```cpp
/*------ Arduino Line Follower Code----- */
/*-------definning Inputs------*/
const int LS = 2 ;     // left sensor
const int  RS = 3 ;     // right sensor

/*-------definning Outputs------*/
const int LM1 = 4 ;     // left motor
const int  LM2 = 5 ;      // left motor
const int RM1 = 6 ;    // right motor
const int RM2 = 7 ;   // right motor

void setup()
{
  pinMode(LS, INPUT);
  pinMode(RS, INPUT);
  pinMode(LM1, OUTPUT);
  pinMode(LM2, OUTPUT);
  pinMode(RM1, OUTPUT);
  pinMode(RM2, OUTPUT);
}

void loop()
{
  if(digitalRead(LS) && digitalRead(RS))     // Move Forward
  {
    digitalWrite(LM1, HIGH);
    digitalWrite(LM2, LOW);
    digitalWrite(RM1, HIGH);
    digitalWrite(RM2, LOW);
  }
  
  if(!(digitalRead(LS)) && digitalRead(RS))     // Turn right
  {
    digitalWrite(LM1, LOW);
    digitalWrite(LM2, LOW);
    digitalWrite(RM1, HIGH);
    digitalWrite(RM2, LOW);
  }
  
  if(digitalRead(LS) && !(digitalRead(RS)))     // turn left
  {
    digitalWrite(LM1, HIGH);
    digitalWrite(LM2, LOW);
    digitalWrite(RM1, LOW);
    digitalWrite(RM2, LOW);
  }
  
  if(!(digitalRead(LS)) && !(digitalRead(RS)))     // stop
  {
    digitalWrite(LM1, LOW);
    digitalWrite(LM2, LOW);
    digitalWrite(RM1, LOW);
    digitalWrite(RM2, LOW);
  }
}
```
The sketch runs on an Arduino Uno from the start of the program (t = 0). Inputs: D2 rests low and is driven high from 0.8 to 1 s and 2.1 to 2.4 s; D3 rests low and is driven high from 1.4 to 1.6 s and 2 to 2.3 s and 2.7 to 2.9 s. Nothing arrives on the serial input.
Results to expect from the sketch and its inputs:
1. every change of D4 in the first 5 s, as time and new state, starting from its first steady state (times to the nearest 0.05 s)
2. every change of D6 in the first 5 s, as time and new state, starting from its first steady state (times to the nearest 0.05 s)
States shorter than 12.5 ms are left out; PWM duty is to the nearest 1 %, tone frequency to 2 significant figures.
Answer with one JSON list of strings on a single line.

["0 s low; 0.8 s high; 1 s low; 2.1 s high; 2.4 s low", "0 s low; 1.4 s high; 1.6 s low; 2 s high; 2.3 s low; 2.7 s high; 2.9 s low"]
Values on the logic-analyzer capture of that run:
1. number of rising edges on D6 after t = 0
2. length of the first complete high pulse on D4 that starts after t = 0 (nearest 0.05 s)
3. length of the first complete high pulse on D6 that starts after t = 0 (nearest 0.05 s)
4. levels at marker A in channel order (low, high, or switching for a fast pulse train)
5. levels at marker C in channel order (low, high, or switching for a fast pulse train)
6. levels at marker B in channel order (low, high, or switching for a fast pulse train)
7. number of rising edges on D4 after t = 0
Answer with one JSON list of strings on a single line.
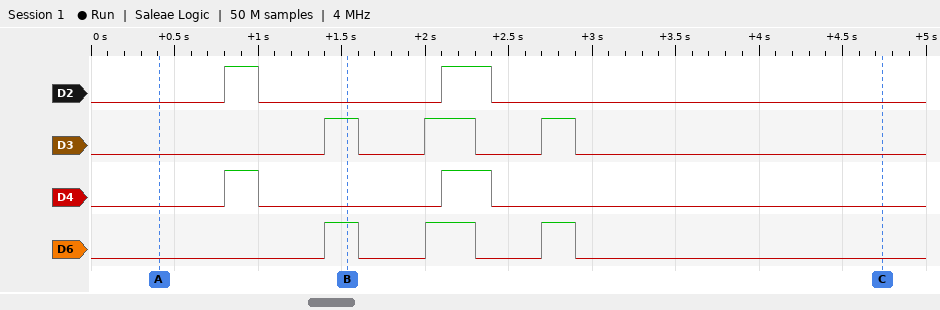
["3", "0.20 s", "0.20 s", "D2 low, D3 low, D4 low, D6 low", "D2 low, D3 low, D4 low, D6 low", "D2 low, D3 high, D4 low, D6 high", "2"]
